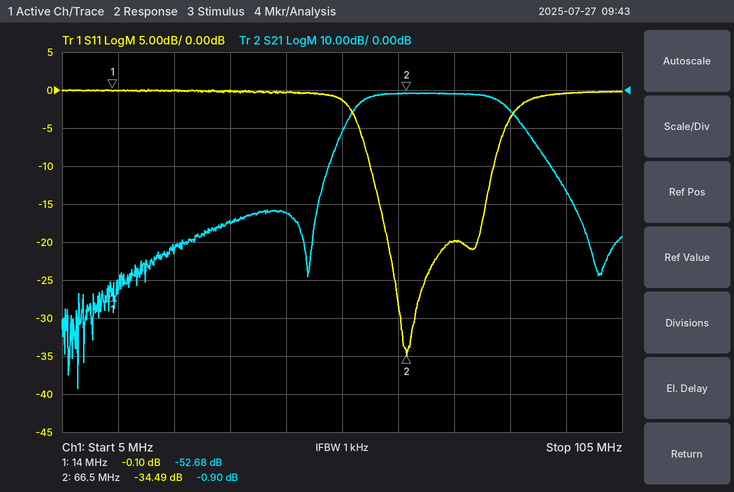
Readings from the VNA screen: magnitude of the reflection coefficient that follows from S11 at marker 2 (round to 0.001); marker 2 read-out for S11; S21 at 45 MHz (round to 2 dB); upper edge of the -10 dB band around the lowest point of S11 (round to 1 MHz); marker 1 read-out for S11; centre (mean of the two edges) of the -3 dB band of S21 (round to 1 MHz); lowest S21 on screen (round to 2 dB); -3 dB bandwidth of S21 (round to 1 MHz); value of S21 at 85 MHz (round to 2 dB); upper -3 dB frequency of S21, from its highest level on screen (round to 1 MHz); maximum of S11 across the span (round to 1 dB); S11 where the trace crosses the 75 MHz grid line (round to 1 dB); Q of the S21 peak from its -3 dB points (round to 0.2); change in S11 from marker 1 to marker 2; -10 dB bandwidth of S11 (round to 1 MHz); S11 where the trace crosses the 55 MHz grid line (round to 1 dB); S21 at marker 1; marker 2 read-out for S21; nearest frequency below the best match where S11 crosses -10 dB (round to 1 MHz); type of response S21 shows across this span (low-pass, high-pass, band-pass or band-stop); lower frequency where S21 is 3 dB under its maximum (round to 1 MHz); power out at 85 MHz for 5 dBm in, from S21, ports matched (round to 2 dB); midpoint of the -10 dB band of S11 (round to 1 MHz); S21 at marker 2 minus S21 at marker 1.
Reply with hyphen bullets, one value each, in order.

- 0.019
- -34.49 dB
- -32 dB
- 82 MHz
- -0.10 dB
- 71 MHz
- -78 dB
- 26 MHz
- -6 dB
- 84 MHz
- 0 dB
- -20 dB
- 2.8
- -34.39 dB
- 22 MHz
- -1 dB
- -52.68 dB
- -0.90 dB
- 60 MHz
- band-pass
- 58 MHz
- 0 dBm
- 71 MHz
- 51.78 dB
